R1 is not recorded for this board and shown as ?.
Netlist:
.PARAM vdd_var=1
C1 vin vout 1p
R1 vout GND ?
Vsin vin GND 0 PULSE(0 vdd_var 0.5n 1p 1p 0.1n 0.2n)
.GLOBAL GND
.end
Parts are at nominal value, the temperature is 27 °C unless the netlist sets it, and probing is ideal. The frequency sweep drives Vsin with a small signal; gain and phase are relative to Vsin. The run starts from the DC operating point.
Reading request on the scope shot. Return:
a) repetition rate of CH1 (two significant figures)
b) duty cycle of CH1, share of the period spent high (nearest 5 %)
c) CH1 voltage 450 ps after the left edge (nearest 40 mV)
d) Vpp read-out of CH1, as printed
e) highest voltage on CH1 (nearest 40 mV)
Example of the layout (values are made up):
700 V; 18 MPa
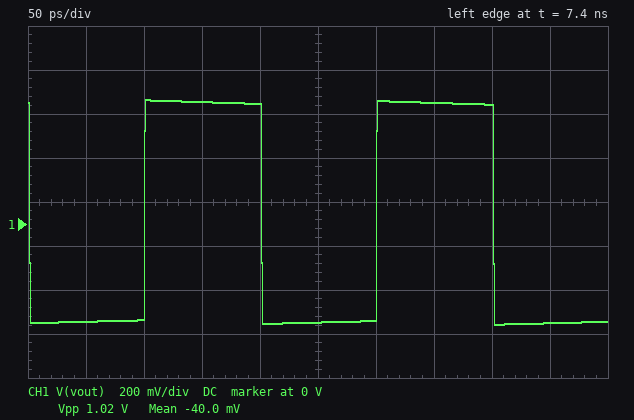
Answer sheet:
5.0 GHz; 50 %; -440 mV; 1.02 V; 560 mV
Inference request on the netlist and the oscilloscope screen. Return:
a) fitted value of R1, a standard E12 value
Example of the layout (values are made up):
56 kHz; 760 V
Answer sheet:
3.3 kΩ
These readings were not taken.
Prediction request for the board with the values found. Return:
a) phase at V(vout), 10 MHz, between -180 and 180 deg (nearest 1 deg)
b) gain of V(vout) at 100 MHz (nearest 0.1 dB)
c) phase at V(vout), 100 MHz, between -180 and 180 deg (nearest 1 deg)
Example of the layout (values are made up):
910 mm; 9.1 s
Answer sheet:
78 deg; -0.9 dB; 26 deg
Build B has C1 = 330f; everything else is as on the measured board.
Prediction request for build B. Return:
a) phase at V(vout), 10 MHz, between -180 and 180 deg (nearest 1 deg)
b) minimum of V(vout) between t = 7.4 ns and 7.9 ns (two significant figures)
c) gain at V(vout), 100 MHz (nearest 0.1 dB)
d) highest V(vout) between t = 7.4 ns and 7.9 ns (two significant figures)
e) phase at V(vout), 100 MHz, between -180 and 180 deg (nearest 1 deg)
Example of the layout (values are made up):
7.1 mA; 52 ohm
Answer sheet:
86 deg; -530 mV; -5.0 dB; 520 mV; 56 deg
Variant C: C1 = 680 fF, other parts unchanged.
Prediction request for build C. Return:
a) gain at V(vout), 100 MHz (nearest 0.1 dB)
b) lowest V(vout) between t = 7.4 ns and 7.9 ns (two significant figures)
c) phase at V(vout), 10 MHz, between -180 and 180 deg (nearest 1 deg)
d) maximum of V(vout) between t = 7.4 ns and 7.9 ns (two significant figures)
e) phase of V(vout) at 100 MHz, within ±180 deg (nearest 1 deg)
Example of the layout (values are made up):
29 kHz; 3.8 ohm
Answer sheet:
-1.8 dB; -500 mV; 82 deg; 530 mV; 35 deg
